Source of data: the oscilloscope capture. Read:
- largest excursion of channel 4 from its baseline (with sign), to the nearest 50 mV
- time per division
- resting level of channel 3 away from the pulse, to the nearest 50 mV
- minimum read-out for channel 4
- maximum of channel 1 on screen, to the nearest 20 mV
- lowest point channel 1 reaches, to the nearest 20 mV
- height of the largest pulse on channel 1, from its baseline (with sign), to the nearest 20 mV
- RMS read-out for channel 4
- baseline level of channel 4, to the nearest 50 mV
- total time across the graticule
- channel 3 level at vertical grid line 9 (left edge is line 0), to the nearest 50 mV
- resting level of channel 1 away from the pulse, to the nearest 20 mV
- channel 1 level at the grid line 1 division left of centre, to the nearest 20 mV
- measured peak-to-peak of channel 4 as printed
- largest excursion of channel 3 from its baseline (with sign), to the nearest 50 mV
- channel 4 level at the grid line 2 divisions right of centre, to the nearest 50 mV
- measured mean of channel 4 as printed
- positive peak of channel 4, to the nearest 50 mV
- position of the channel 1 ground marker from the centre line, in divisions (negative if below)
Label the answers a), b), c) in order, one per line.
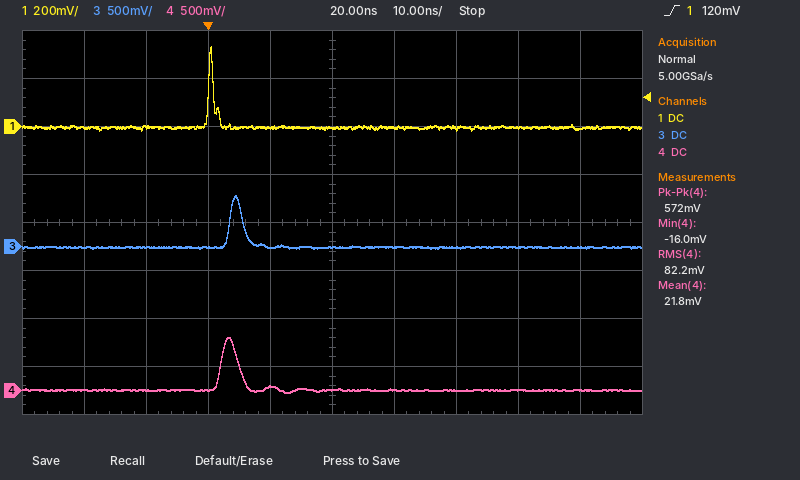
a) +550 mV
b) 10 ns
c) 0 mV
d) -16.0 mV
e) 340 mV
f) -20 mV
g) +340 mV
h) 82.2 mV
i) 0 mV
j) 100 ns
k) 0 mV
l) 0 mV
m) 0 mV
n) 572 mV
o) +550 mV
p) 0 mV
q) 21.8 mV
r) 550 mV
s) +2.0 div
